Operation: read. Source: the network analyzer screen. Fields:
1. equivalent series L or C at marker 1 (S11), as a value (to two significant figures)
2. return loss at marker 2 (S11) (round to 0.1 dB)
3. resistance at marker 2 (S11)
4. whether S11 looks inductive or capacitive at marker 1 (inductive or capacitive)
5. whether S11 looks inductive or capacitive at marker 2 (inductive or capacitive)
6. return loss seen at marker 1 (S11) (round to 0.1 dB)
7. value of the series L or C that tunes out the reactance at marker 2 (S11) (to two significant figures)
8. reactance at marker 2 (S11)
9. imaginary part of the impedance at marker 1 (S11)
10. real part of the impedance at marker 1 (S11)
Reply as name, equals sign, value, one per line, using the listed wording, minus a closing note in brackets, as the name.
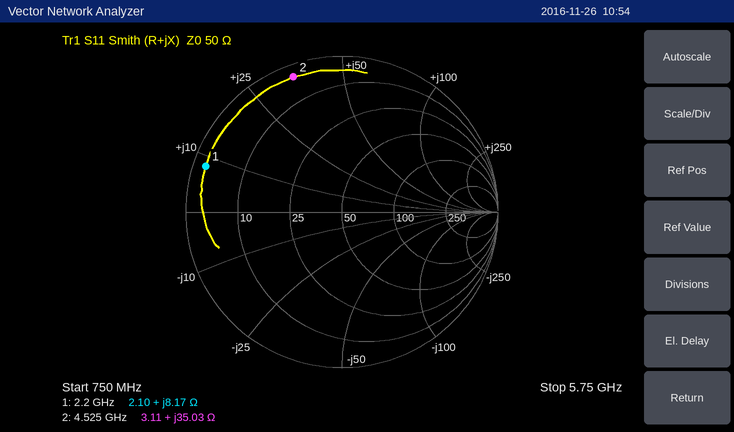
equivalent series L or C at marker 1 (S11), as a value = 590 pH
return loss at marker 2 (S11) = 0.7 dB
resistance at marker 2 = 3.11 Ω
whether S11 looks inductive or capacitive at marker 1 = inductive
whether S11 looks inductive or capacitive at marker 2 = inductive
return loss seen at marker 1 (S11) = 0.7 dB
value of the series L or C that tunes out the reactance at marker 2 (S11) = 1.0 pF
reactance at marker 2 = +35.03 Ω
imaginary part of the impedance at marker 1 = +8.17 Ω
real part of the impedance at marker 1 = 2.10 Ω
